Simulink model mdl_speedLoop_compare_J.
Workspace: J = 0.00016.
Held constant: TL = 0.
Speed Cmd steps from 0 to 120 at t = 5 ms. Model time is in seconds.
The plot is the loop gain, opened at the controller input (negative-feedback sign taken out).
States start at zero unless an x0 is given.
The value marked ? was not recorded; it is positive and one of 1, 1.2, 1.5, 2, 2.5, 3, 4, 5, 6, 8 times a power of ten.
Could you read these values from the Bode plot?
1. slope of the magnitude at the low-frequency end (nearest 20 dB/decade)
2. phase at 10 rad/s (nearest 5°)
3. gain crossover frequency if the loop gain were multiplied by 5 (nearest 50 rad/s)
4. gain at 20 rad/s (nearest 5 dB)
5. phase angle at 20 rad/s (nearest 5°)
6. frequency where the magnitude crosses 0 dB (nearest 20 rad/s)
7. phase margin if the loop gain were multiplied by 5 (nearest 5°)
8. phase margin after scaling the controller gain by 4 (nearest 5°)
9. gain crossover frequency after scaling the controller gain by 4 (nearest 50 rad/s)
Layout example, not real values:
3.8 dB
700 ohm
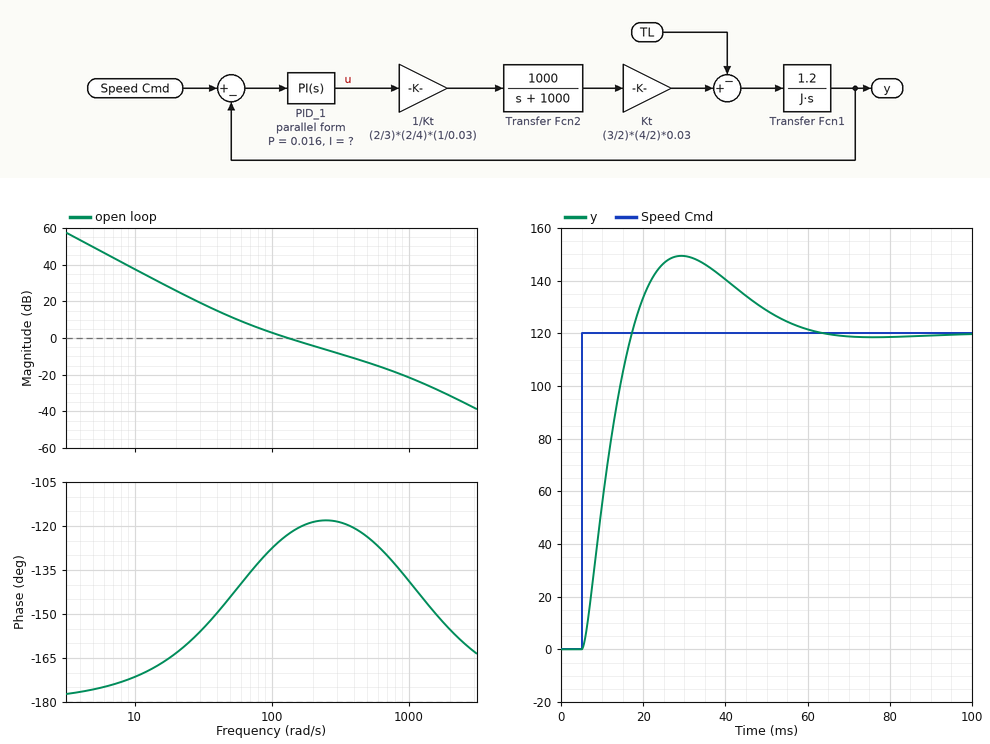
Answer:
-40 dB/decade
-170°
550 rad/s
25 dB
-165°
140 rad/s
55°
60°
450 rad/s
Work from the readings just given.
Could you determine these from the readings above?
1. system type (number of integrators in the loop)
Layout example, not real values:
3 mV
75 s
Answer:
2
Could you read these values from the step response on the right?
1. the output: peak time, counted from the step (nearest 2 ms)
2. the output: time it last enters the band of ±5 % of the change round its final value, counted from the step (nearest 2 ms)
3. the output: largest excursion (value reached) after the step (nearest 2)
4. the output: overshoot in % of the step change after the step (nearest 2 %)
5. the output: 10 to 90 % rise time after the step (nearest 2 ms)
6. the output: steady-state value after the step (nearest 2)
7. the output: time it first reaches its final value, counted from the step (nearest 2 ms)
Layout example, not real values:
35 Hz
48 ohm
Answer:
24 ms
48 ms
150
24 %
8 ms
120
12 ms
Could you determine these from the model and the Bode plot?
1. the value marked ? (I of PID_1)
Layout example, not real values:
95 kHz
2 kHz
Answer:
1
